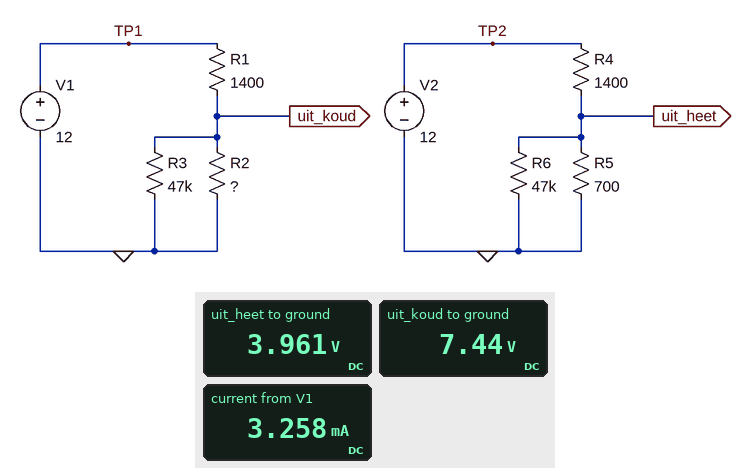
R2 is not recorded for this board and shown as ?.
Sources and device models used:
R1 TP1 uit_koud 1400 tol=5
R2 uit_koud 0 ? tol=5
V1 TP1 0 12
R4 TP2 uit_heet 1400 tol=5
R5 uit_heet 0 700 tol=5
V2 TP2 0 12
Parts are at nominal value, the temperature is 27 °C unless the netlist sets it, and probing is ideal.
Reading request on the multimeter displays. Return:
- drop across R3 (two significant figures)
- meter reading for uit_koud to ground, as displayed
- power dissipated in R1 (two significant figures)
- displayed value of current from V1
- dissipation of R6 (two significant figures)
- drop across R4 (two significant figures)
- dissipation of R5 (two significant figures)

7.4 V
7.44 V
15 mW
3.258 mA
330 µW
8.0 V
22 mW
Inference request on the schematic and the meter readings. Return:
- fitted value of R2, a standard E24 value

2.4 kΩ
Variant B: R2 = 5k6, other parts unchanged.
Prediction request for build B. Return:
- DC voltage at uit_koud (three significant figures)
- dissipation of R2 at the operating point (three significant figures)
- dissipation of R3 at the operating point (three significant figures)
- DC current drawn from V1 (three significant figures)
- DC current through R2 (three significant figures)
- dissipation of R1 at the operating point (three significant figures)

9.38 V
15.7 mW
1.87 mW
1.87 mA
1.67 mA
4.92 mW
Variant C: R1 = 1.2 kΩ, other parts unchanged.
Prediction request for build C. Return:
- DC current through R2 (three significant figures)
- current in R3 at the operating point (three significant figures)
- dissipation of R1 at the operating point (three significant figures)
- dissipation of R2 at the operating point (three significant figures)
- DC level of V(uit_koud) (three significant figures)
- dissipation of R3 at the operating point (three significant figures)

3.28 mA
167 µA
14.2 mW
25.8 mW
7.87 V
1.32 mW
